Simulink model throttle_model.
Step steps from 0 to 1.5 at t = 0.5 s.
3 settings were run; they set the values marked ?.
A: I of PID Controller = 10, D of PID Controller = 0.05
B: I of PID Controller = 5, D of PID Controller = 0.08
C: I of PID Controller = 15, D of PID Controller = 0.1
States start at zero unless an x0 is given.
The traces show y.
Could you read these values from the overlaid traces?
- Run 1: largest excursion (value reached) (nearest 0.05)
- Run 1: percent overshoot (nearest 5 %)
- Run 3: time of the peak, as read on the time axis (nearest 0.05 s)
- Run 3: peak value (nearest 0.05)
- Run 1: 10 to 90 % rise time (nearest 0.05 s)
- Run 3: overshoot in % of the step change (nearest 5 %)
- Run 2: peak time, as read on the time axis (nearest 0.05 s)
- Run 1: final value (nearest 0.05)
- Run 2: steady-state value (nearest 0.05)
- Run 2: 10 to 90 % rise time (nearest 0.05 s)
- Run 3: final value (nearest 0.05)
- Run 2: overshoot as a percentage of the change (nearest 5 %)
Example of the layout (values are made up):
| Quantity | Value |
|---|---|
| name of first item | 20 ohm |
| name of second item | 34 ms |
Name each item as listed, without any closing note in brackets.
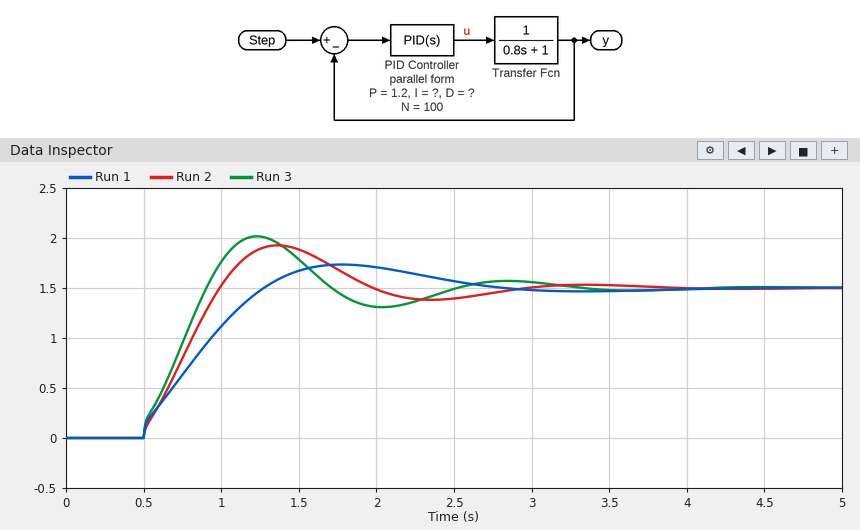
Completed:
| Quantity | Value |
|---|---|
| Run 1: largest excursion (value reached) | 1.75 |
| Run 1: percent overshoot | 15 % |
| Run 3: time of the peak, as read on the time axis | 1.25 s |
| Run 3: peak value | 2.00 |
| Run 1: 10 to 90 % rise time | 0.65 s |
| Run 3: overshoot in % of the step change | 35 % |
| Run 2: peak time, as read on the time axis | 1.35 s |
| Run 1: final value | 1.50 |
| Run 2: steady-state value | 1.50 |
| Run 2: 10 to 90 % rise time | 0.40 s |
| Run 3: final value | 1.50 |
| Run 2: overshoot as a percentage of the change | 30 % |
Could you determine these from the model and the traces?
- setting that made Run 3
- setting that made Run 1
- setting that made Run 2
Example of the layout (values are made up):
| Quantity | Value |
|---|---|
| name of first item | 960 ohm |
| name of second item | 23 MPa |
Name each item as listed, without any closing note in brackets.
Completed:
| Quantity | Value |
|---|---|
| setting that made Run 3 | C |
| setting that made Run 1 | B |
| setting that made Run 2 | A |
